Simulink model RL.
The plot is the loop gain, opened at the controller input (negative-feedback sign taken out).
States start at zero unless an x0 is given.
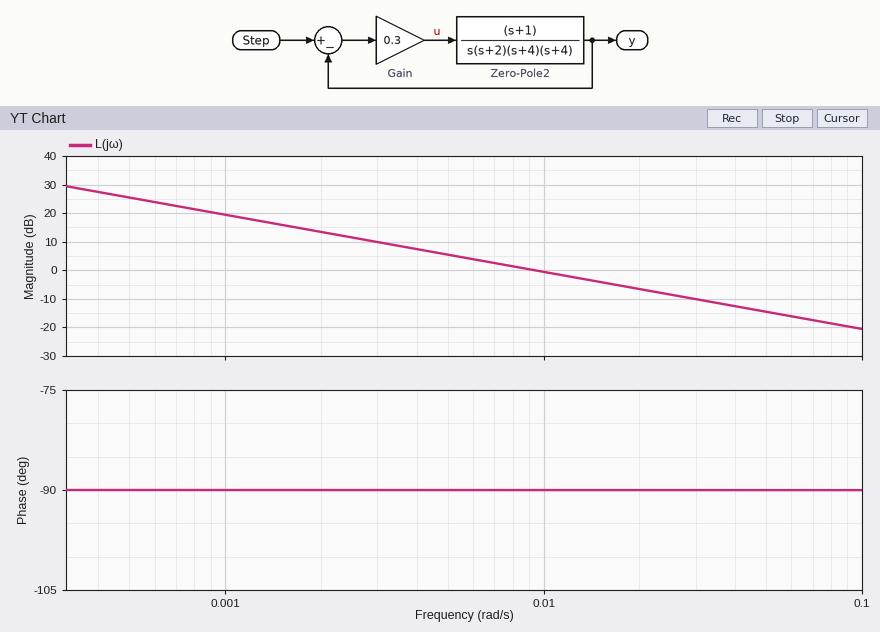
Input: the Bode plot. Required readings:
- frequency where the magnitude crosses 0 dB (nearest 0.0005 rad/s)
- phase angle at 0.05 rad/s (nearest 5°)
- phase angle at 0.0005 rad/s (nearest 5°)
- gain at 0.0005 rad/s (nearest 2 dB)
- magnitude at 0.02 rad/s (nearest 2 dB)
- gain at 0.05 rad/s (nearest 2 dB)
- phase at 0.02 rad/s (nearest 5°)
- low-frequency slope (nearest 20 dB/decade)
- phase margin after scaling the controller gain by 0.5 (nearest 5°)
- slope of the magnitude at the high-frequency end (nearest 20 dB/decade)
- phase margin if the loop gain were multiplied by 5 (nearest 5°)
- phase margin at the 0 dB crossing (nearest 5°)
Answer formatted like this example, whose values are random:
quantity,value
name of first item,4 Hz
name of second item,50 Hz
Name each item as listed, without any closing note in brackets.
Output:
quantity,value
frequency where the magnitude crosses 0 dB,0.0095 rad/s
phase angle at 0.05 rad/s,-90°
phase angle at 0.0005 rad/s,-90°
gain at 0.0005 rad/s,26 dB
magnitude at 0.02 rad/s,-6 dB
gain at 0.05 rad/s,-14 dB
phase at 0.02 rad/s,-90°
low-frequency slope,-20 dB/decade
phase margin after scaling the controller gain by 0.5,90°
slope of the magnitude at the high-frequency end,-20 dB/decade
phase margin if the loop gain were multiplied by 5,90°
phase margin at the 0 dB crossing,90°
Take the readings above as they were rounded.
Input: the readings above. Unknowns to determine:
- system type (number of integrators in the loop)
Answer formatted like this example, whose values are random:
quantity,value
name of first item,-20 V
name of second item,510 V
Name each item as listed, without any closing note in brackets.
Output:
quantity,value
system type,1
